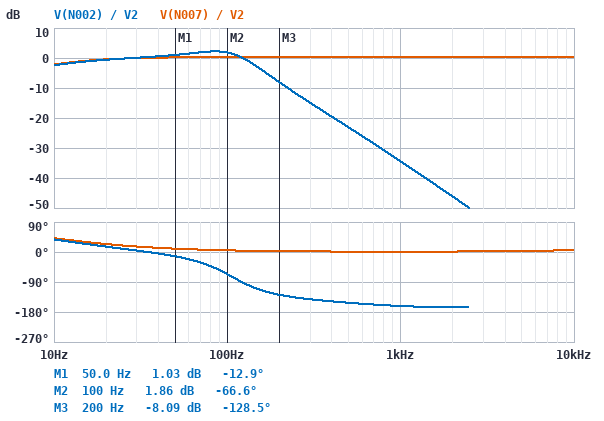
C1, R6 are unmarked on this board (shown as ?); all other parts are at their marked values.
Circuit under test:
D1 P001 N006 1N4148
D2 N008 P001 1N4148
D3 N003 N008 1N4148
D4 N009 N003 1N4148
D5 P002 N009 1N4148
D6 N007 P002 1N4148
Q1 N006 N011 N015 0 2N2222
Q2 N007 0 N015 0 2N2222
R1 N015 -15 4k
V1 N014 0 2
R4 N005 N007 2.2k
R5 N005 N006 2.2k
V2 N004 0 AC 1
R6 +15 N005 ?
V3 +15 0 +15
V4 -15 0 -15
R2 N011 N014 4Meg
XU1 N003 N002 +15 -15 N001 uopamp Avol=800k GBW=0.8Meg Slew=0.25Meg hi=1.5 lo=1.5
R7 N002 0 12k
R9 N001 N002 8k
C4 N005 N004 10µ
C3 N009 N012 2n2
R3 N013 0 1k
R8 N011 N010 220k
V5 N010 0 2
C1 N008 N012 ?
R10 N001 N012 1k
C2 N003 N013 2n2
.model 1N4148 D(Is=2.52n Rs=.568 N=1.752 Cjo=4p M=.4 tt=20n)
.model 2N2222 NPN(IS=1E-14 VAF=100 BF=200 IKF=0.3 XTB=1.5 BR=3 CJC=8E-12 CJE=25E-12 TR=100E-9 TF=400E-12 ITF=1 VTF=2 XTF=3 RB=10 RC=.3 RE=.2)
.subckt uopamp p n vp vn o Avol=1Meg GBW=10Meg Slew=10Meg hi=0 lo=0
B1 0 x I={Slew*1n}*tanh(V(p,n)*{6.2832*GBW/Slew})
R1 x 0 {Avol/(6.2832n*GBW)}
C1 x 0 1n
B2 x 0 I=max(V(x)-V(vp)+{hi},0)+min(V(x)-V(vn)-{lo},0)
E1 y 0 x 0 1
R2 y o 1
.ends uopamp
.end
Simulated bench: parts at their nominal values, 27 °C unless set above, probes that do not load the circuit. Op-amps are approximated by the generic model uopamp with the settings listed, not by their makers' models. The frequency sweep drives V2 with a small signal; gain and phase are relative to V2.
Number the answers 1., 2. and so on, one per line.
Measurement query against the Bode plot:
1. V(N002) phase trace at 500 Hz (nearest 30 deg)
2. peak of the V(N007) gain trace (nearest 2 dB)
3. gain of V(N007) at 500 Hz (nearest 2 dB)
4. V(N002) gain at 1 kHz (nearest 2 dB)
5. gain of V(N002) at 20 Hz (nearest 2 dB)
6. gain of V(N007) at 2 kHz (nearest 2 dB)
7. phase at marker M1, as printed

1. -150 deg
2. 0 dB
3. 0 dB
4. -34 dB
5. 0 dB
6. 0 dB
7. -12.9 deg
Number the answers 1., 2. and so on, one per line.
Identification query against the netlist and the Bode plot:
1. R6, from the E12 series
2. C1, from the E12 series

1. 1.8 kΩ
2. 680 pF
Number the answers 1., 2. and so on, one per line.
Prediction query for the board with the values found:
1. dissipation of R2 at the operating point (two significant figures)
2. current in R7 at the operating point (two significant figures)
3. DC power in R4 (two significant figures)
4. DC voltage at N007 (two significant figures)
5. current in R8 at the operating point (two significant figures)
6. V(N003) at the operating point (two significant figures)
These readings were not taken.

1. 990 nW
2. 390 µA
3. 5.5 mW
4. 5.1 V
5. 9.1 µA
6. 4.7 V
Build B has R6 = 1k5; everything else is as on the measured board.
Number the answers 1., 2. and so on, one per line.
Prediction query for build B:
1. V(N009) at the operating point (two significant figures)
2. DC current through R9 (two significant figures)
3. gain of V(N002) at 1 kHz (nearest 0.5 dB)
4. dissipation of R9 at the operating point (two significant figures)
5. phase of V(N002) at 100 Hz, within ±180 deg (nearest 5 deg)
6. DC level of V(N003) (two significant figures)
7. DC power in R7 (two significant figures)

1. 5.9 V
2. 480 µA
3. -29.5 dB
4. 1.8 mW
5. -35 deg
6. 5.7 V
7. 2.7 mW
